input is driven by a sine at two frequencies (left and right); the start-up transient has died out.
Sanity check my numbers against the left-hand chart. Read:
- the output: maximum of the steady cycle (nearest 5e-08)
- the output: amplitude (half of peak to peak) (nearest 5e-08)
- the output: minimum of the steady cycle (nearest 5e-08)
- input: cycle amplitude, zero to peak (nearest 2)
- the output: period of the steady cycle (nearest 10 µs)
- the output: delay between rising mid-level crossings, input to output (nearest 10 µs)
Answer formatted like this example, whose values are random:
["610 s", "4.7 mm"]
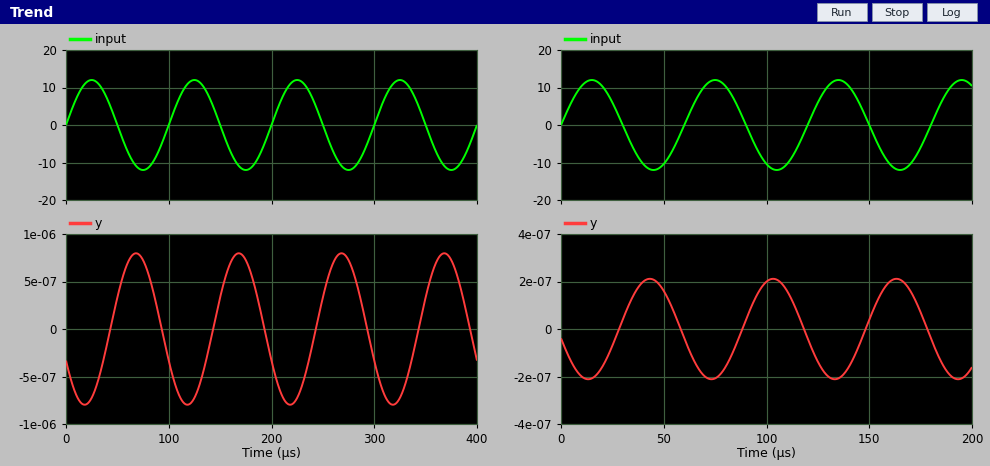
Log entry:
["0.00000080", "0.00000080", "-0.00000080", "12", "100 µs", "40 µs"]
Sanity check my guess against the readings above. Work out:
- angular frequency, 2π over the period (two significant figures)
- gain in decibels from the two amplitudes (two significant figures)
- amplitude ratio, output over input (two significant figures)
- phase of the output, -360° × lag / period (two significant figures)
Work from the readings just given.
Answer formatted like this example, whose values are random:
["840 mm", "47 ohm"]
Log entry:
["0.063 rad/µs", "-140 dB", "0.000000067", "-140°"]
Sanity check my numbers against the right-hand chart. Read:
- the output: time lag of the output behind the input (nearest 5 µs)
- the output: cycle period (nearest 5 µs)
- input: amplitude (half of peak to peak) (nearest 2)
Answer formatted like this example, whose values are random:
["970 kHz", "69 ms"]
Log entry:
["30 µs", "60 µs", "12"]
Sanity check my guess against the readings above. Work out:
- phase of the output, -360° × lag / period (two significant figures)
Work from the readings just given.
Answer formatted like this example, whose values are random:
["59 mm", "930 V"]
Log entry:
["-180°"]
